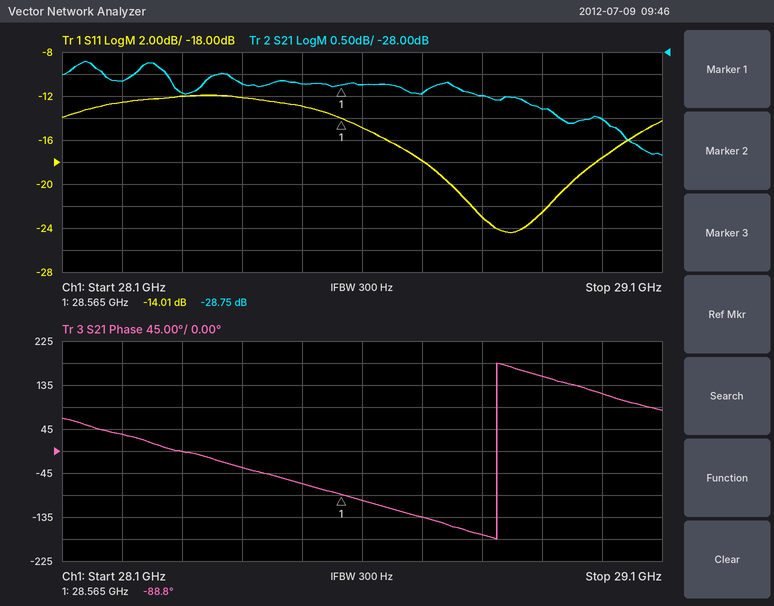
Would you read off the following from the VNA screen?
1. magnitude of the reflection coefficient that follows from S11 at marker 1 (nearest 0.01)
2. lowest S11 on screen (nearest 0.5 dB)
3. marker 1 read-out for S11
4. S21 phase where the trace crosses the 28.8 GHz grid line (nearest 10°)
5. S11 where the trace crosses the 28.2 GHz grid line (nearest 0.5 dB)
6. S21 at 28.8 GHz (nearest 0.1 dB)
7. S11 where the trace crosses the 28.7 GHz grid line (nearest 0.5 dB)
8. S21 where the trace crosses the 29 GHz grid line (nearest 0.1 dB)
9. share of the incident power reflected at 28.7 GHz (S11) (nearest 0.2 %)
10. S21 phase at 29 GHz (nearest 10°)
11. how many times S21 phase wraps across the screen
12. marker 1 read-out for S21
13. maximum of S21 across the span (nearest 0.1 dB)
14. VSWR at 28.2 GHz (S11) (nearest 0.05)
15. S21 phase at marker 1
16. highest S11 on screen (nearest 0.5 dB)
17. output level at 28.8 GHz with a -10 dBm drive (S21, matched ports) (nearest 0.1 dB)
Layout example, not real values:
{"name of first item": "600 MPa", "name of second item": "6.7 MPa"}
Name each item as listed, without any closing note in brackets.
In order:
{"magnitude of the reflection coefficient that follows from S11 at marker 1": "0.20", "lowest S11 on screen": "-24.5 dB", "marker 1 read-out for S11": "-14.01 dB", "S21 phase where the trace crosses the 28.8 GHz grid line": "-170°", "S11 where the trace crosses the 28.2 GHz grid line": "-12.5 dB", "S21 at 28.8 GHz": "-29.0 dB", "S11 where the trace crosses the 28.7 GHz grid line": "-18.0 dB", "S21 where the trace crosses the 29 GHz grid line": "-29.5 dB", "share of the incident power reflected at 28.7 GHz (S11)": "1.6 %", "S21 phase at 29 GHz": "120°", "how many times S21 phase wraps across the screen": "1", "marker 1 read-out for S21": "-28.75 dB", "maximum of S21 across the span": "-28.2 dB", "VSWR at 28.2 GHz (S11)": "1.60", "S21 phase at marker 1": "-88.8°", "highest S11 on screen": "-12.0 dB", "output level at 28.8 GHz with a -10 dBm drive (S21, matched ports)": "-39.0 dBm"}
